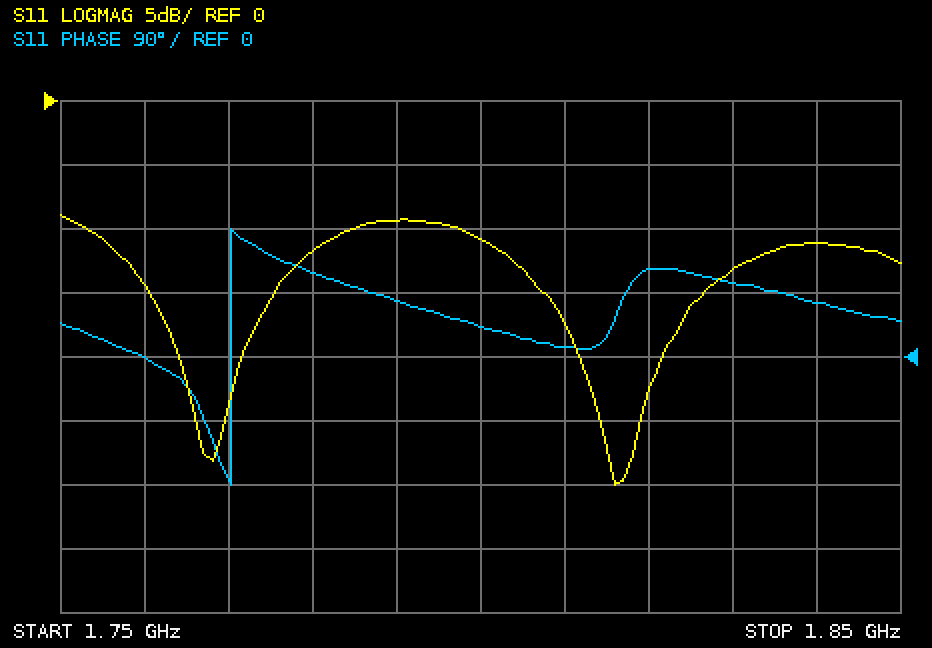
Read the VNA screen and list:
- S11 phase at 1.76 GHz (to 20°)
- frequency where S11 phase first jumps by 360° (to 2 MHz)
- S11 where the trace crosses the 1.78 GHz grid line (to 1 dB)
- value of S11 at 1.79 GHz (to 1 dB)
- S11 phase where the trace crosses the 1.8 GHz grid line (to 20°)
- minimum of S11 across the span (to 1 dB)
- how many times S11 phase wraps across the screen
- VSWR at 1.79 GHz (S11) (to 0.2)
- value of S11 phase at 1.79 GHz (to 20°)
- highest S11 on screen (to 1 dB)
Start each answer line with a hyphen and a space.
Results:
- 0°
- 1.770 GHz
- -12 dB
- -9 dB
- 40°
- -30 dB
- 1
- 2.0
- 80°
- -9 dB
